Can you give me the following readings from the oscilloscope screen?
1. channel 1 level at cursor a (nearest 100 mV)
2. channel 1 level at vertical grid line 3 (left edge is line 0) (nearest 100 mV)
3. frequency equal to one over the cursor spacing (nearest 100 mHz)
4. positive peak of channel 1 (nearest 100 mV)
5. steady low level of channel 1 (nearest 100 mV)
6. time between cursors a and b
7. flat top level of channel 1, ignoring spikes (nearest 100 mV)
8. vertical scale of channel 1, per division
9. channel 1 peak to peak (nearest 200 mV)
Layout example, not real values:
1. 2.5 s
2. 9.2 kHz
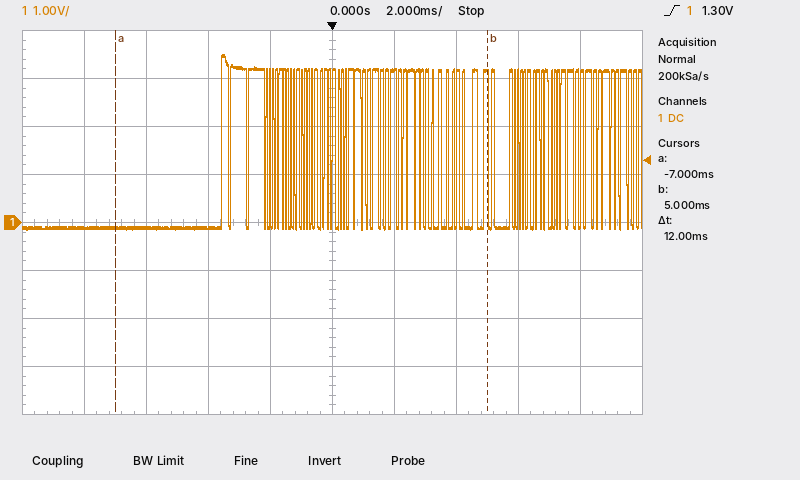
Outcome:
1. -100 mV
2. -100 mV
3. 83.3 Hz
4. 3.5 V
5. -100 mV
6. 12 ms
7. 3.2 V
8. 1 V
9. 3.6 V
